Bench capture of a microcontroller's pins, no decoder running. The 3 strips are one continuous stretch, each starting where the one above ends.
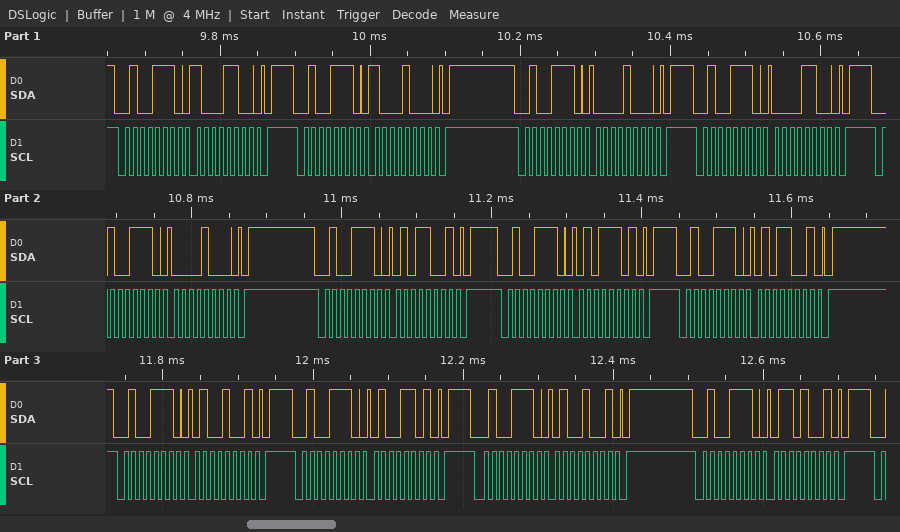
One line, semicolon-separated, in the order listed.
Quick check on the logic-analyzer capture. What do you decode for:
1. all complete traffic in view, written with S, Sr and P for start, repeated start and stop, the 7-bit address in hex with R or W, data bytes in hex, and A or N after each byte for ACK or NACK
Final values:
S 27W A 8C A P S 27W A 88 A P S 27W A 08 A P S 27W A 0C A P S 27W A 08 A P S 27W A 59 A P S 27W A 5D A P S 27W A 59 A P S 27W A 49 A P S 27W A 4D A P S 27W A 49 A P S 27W A 69 A P
